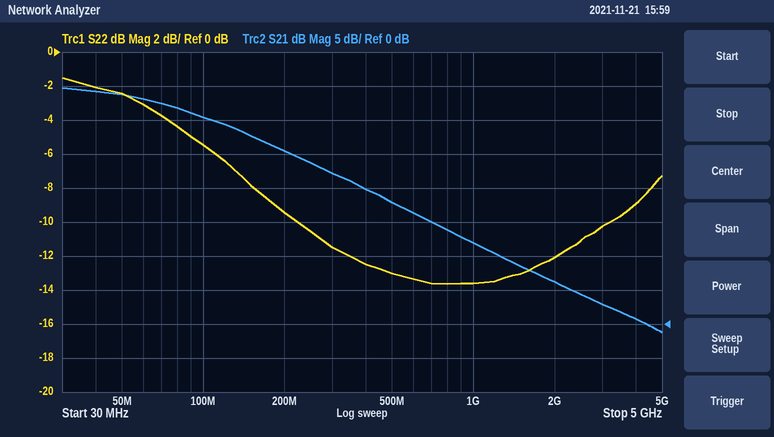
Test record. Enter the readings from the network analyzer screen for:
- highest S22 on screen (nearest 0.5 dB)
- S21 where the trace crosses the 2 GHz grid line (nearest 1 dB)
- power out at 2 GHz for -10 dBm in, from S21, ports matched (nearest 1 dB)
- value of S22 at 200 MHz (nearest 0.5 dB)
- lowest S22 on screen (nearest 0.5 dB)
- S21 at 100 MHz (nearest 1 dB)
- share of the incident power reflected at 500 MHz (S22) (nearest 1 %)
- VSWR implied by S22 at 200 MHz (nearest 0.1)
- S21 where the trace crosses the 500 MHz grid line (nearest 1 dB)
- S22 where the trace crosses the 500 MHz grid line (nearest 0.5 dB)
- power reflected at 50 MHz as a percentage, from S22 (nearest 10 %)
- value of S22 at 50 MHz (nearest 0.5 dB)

-1.5 dB
6 dB
-4 dBm
-9.5 dB
-13.5 dB
30 dB
5 %
2.0
18 dB
-13.0 dB
60 %
-2.5 dB
